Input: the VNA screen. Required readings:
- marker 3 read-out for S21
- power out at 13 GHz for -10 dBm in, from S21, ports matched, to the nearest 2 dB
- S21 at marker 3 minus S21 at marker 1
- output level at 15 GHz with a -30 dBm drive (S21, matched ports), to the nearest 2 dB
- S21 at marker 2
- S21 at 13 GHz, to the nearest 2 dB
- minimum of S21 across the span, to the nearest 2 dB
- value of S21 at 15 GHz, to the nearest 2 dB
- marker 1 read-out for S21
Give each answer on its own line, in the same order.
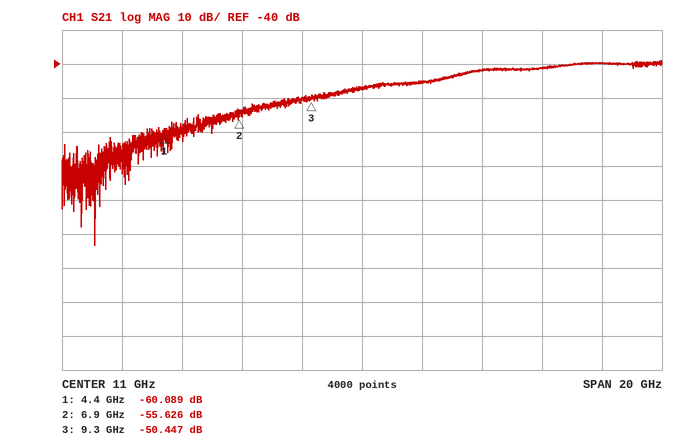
-50.447 dB
-56 dBm
9.642 dB
-72 dBm
-55.626 dB
-46 dB
-94 dB
-42 dB
-60.089 dB
